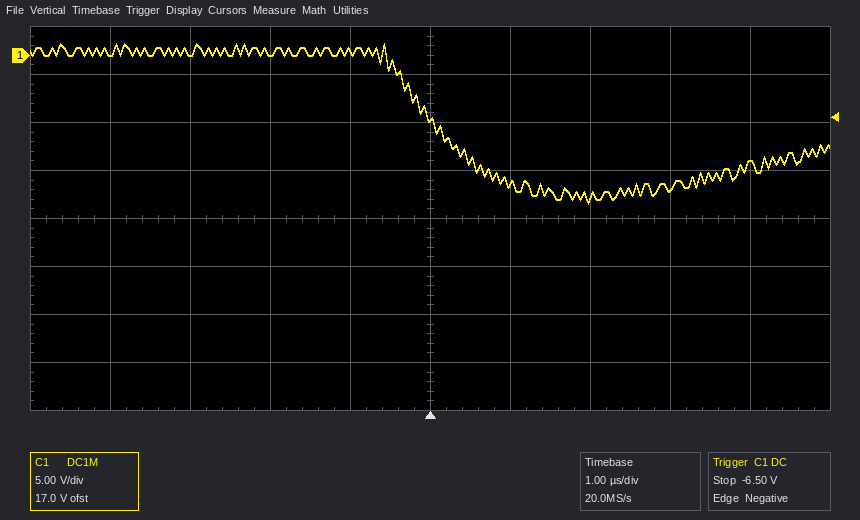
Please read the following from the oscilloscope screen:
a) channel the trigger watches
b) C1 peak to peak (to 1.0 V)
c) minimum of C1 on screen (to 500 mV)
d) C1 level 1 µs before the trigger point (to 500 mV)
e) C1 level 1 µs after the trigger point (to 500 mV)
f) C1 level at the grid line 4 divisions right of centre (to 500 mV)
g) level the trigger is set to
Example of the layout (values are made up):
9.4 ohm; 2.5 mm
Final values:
C1; 17.0 V; -15.5 V; 500 mV; -13.5 V; -11.5 V; -6.50 V
